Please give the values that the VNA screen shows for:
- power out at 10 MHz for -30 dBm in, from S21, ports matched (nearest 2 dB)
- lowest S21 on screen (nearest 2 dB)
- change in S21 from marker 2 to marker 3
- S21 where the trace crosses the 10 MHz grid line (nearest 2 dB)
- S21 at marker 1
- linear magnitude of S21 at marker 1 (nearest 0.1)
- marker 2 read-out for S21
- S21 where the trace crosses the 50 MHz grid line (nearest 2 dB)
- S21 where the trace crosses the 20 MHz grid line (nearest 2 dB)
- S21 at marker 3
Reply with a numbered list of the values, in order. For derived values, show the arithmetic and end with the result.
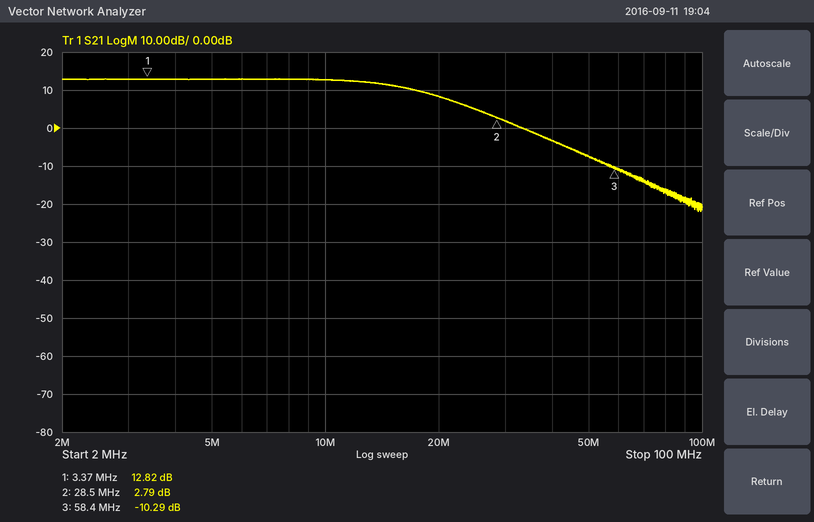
1. -30 dBm + (12 dB) = -18 dBm
2. -22 dB
3. -10.29 − (2.79) = -13.08 dB
4. 12 dB
5. 12.82 dB
6. 10^(12.82/20) ≈ 4.4
7. 2.79 dB
8. -8 dB
9. 8 dB
10. -10.29 dB
